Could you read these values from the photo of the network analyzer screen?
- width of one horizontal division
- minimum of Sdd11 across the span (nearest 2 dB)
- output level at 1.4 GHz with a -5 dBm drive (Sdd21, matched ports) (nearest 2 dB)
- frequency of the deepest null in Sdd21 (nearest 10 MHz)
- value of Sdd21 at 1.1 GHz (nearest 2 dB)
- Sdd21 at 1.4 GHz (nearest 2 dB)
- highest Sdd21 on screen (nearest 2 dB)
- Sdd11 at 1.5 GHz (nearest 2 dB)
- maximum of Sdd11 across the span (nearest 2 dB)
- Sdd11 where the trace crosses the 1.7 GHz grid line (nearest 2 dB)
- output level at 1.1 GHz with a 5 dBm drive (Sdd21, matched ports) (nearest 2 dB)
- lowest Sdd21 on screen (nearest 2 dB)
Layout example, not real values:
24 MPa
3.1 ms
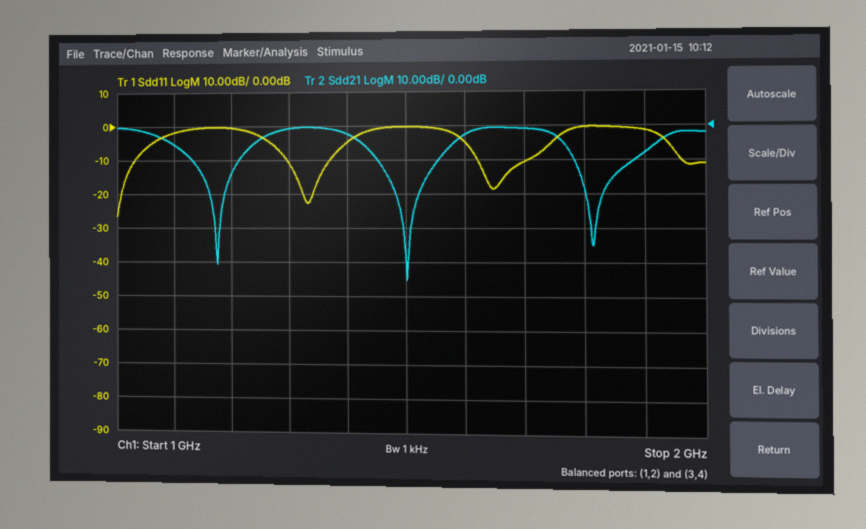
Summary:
100 MHz
-26 dB
-8 dBm
1.50 GHz
-6 dB
-2 dB
0 dB
0 dB
0 dB
-10 dB
0 dBm
-46 dB
